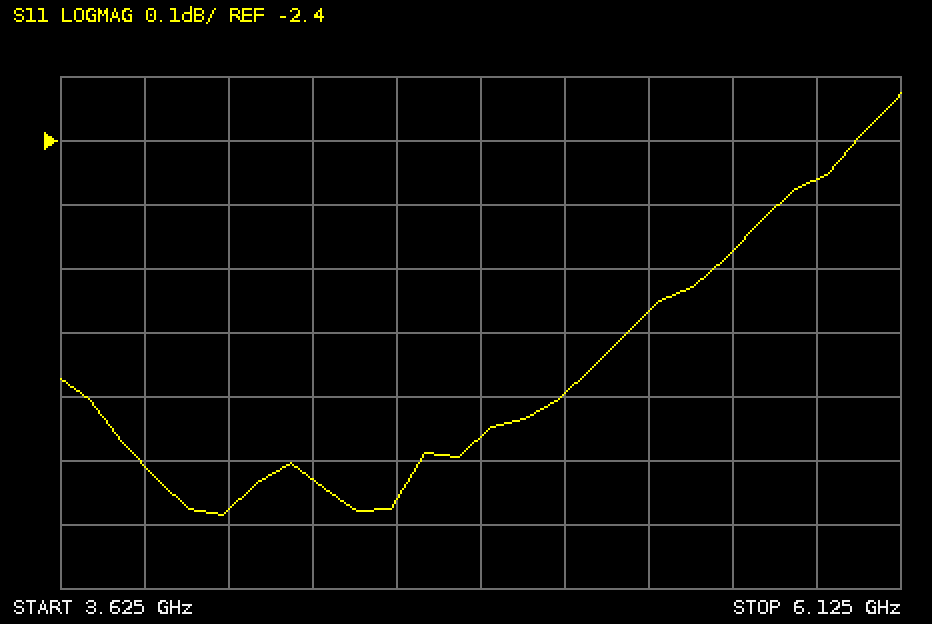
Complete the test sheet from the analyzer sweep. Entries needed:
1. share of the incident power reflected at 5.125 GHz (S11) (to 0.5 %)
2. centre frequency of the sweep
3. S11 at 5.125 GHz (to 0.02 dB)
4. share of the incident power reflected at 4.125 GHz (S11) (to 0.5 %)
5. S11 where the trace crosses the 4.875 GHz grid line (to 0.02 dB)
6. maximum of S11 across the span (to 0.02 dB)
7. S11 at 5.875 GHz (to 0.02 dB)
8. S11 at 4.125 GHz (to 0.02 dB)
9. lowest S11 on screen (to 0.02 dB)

52.5 %
4.875 GHz
-2.80 dB
50.5 %
-2.86 dB
-2.32 dB
-2.46 dB
-2.98 dB
-2.98 dB
